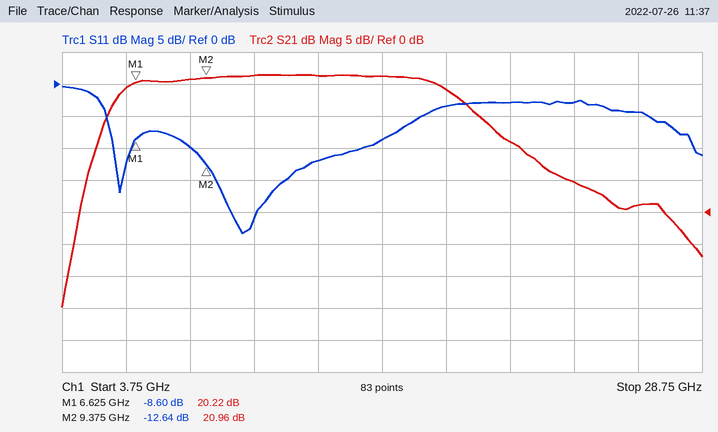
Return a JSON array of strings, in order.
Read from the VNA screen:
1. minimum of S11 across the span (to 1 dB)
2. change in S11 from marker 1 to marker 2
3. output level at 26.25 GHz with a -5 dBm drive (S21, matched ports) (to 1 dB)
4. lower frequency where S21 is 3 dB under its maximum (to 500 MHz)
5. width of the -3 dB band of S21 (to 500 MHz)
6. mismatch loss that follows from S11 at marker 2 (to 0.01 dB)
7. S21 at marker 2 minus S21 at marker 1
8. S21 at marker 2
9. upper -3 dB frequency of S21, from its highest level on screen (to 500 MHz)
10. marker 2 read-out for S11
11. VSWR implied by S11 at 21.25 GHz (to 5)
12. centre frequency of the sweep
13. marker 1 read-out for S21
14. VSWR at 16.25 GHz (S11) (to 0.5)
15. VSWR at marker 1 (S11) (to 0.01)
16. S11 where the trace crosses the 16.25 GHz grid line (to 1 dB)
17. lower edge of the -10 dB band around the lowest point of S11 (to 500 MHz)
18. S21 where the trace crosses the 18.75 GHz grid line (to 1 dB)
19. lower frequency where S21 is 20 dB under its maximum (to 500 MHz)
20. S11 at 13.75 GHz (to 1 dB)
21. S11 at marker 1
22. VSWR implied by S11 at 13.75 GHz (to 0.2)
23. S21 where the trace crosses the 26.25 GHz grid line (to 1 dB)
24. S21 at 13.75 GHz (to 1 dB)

["-23 dB", "-4.04 dB", "-4 dBm", "6.0 GHz", "13.0 GHz", "0.24 dB", "0.74 dB", "20.96 dB", "19.0 GHz", "-12.64 dB", "5", "16.25 GHz", "20.22 dB", "2.0", "2.18", "-9 dB", "9.0 GHz", "19 dB", "4.5 GHz", "-12 dB", "-8.60 dB", "1.6", "1 dB", "21 dB"]
